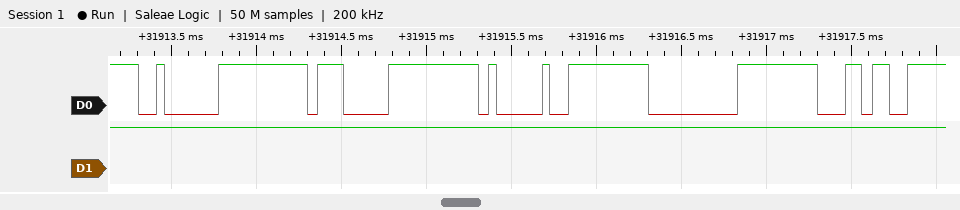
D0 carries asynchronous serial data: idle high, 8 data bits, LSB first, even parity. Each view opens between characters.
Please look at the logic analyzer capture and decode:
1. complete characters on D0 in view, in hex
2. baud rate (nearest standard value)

02, 07, 41, 00, 6C
19200 baud
